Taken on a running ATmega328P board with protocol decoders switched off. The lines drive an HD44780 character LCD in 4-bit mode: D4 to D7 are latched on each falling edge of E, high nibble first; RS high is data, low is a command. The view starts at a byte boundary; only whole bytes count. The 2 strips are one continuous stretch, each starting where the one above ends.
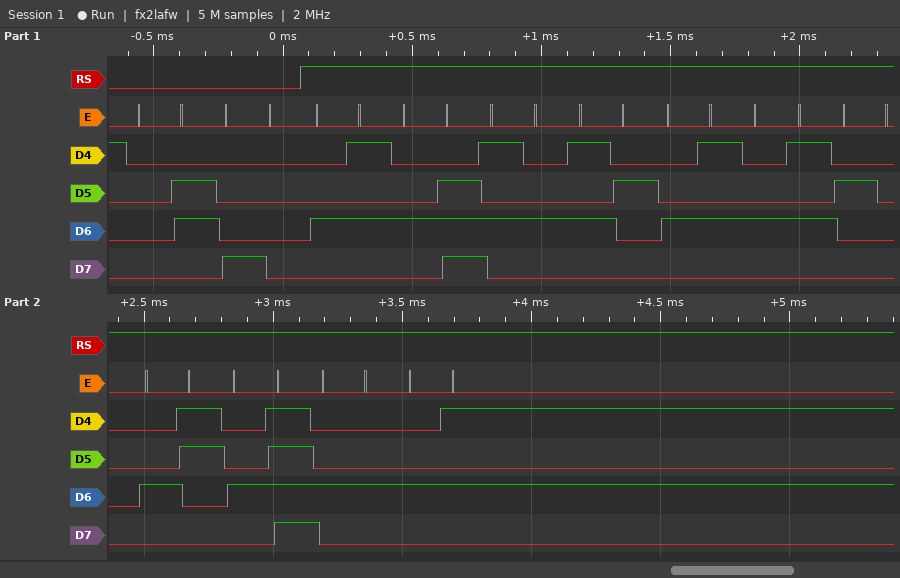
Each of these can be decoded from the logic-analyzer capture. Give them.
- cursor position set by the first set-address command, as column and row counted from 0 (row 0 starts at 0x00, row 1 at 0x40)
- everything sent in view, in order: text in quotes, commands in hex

column 0, row 0
0x06 0x80 "ENTREE CODE"
